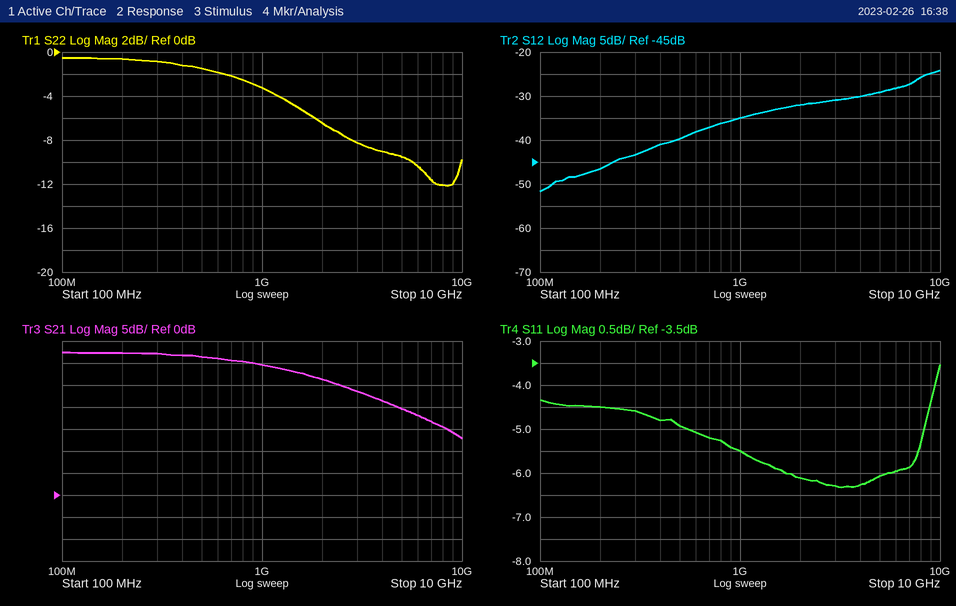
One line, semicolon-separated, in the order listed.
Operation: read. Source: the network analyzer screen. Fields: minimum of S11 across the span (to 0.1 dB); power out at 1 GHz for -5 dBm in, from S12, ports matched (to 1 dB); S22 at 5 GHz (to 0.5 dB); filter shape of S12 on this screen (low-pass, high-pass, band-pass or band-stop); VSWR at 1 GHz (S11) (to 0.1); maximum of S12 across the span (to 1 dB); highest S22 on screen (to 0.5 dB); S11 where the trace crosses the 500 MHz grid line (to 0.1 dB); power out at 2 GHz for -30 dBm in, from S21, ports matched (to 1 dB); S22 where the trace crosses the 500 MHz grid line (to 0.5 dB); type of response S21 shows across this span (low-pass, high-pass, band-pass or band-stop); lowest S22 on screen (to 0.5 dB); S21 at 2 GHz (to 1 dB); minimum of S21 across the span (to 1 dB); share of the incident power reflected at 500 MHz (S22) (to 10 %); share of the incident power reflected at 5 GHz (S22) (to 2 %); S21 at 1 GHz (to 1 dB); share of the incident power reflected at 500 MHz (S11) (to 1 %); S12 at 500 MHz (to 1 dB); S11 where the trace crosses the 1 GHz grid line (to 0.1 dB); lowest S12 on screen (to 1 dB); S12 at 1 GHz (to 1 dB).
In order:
-6.3 dB; -40 dBm; -9.5 dB; high-pass; 3.3; -24 dB; -0.5 dB; -4.9 dB; -4 dBm; -1.5 dB; low-pass; -12.0 dB; 26 dB; 13 dB; 70 %; 12 %; 30 dB; 32 %; -40 dB; -5.5 dB; -52 dB; -35 dB
